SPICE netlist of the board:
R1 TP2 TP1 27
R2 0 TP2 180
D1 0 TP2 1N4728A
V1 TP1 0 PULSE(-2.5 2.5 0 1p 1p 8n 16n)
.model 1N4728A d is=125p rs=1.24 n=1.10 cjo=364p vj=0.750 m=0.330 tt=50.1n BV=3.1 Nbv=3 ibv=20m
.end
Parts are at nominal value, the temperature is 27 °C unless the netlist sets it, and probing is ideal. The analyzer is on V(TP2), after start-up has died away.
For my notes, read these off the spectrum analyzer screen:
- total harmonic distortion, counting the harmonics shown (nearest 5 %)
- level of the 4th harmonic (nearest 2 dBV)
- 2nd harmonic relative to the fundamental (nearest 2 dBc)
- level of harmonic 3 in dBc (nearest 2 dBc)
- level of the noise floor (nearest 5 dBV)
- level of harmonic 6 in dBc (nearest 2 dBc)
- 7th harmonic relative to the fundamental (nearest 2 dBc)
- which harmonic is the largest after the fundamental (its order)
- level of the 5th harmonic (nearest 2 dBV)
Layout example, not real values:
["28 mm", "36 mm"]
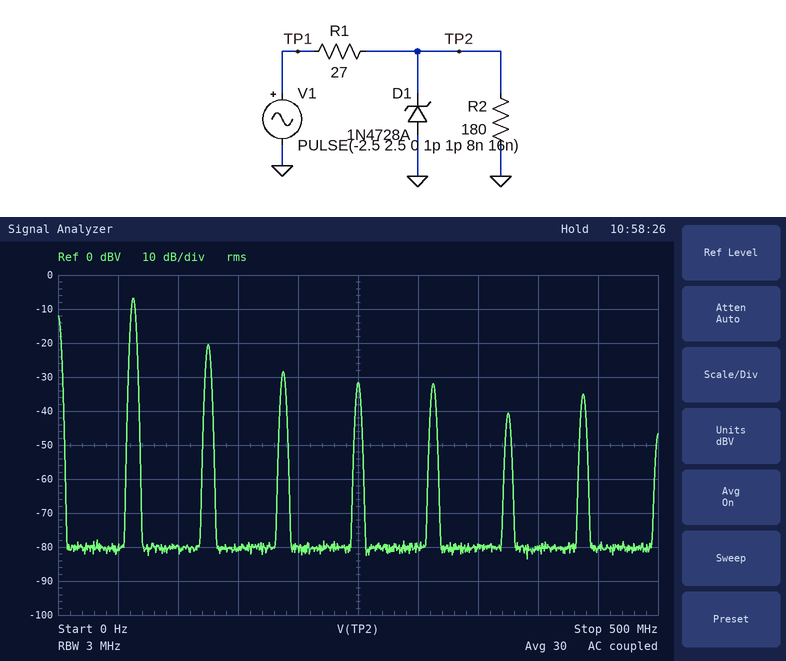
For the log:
["25 %", "-32 dBV", "-14 dBc", "-22 dBc", "-80 dBV", "-34 dBc", "-28 dBc", "2", "-32 dBV"]
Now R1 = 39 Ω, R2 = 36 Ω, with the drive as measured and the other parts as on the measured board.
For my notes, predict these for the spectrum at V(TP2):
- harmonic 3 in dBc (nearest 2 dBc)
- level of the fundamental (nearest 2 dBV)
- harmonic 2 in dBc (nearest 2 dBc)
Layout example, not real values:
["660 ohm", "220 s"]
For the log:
["-20 dBc", "-10 dBV", "-20 dBc"]
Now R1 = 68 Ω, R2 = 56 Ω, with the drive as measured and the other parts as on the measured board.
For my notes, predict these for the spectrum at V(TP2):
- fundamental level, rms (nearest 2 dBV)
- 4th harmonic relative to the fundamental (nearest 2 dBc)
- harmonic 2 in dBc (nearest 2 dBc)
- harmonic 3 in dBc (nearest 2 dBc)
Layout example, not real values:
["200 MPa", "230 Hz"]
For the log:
["-14 dBV", "-40 dBc", "-28 dBc", "-18 dBc"]
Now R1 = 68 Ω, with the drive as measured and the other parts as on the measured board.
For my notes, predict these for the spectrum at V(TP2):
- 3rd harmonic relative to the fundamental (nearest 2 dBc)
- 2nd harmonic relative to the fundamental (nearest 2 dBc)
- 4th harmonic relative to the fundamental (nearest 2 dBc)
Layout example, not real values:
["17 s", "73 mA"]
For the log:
["-18 dBc", "-28 dBc", "-38 dBc"]
